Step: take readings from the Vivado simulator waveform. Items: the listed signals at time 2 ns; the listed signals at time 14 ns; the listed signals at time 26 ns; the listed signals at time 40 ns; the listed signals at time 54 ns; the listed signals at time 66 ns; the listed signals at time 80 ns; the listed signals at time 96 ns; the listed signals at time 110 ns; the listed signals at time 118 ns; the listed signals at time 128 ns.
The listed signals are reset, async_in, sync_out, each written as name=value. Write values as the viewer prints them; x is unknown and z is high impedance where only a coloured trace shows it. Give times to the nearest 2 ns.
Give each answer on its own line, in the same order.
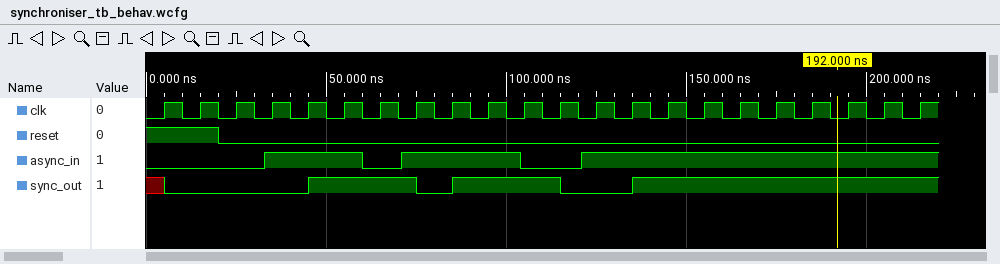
reset=1, async_in=0, sync_out=x
reset=1, async_in=0, sync_out=0
reset=0, async_in=0, sync_out=0
reset=0, async_in=1, sync_out=0
reset=0, async_in=1, sync_out=1
reset=0, async_in=0, sync_out=1
reset=0, async_in=1, sync_out=0
reset=0, async_in=1, sync_out=1
reset=0, async_in=0, sync_out=1
reset=0, async_in=0, sync_out=0
reset=0, async_in=1, sync_out=0
